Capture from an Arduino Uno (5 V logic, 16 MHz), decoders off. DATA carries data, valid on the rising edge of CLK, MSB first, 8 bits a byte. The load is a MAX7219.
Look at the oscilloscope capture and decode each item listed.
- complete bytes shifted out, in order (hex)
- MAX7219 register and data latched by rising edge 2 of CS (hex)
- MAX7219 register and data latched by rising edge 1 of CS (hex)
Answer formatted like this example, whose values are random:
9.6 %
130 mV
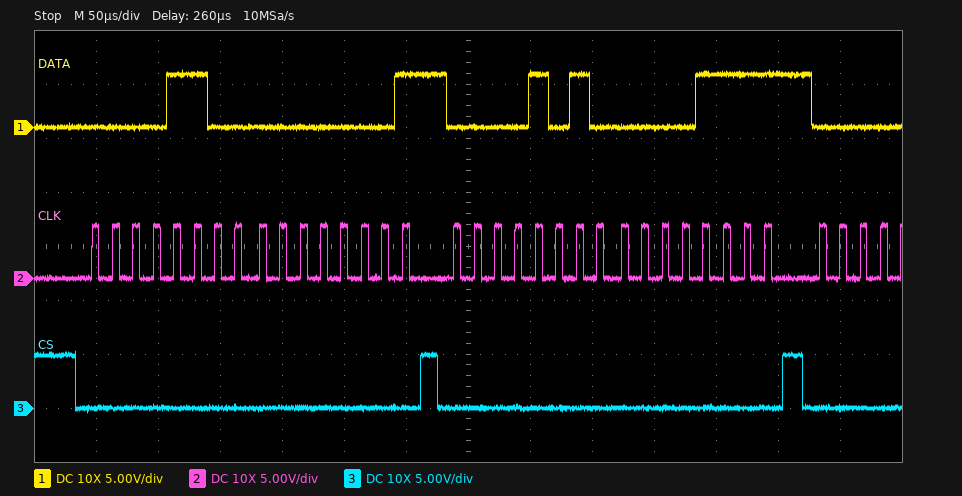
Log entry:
0C 01 0A 0F
register 0xA, data 0x0F
register 0xC, data 0x01
